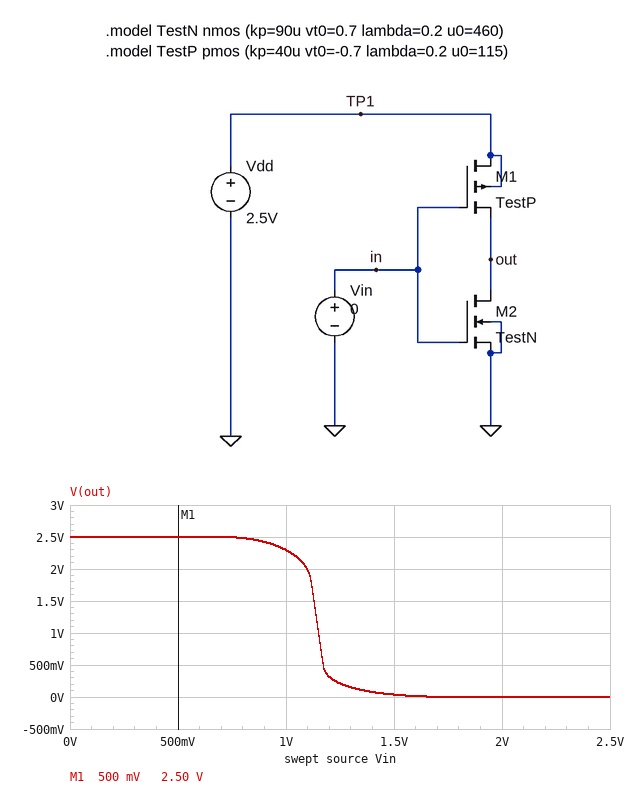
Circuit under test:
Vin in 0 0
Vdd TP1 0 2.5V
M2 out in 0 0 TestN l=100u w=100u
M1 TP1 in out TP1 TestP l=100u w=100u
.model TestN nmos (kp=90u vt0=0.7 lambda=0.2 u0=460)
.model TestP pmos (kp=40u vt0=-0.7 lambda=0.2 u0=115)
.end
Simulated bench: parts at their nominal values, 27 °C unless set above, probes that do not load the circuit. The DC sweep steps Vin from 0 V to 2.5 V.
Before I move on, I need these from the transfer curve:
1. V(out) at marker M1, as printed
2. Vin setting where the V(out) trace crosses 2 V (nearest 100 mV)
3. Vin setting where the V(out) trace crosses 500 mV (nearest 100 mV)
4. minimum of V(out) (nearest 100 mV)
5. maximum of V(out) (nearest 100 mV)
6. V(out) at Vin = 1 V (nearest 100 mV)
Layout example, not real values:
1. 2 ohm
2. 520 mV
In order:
1. 2.50 V
2. 1.1 V
3. 1.2 V
4. 0 V
5. 2.5 V
6. 2.3 V
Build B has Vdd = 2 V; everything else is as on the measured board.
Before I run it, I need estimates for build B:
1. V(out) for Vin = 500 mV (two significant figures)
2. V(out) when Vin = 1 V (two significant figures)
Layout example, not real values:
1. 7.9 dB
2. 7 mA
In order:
1. 2.0 V
2. 110 mV
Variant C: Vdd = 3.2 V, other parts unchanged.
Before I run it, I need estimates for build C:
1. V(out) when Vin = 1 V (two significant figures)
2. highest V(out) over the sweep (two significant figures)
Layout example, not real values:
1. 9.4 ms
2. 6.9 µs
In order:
1. 3.1 V
2. 3.2 V
